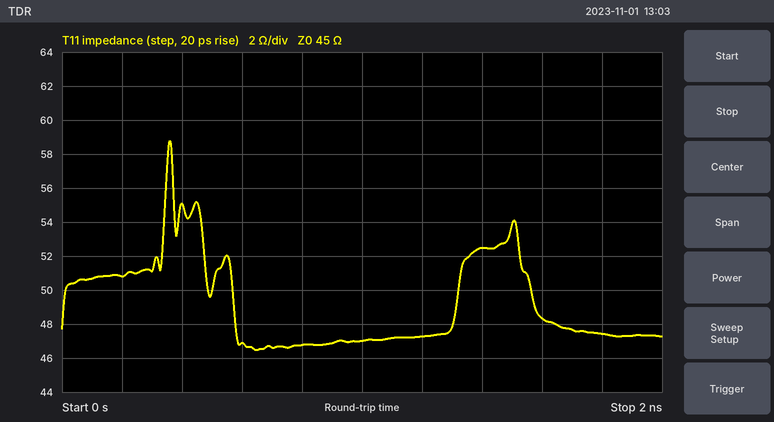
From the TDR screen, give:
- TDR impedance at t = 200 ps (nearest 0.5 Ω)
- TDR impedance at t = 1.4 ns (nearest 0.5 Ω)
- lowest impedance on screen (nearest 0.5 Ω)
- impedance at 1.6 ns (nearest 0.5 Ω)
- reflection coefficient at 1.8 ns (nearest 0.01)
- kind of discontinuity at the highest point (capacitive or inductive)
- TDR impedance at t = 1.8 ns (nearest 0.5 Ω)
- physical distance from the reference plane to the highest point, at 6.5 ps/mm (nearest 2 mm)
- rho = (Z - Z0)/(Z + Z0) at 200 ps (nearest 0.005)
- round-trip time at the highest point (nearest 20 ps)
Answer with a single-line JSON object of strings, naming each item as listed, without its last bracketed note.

{"TDR impedance at t = 200 ps": "51.0 Ω", "TDR impedance at t = 1.4 ns": "52.5 Ω", "lowest impedance on screen": "46.5 Ω", "impedance at 1.6 ns": "48.5 Ω", "reflection coefficient at 1.8 ns": "+0.03", "kind of discontinuity at the highest point": "inductive", "TDR impedance at t = 1.8 ns": "47.5 Ω", "physical distance from the reference plane to the highest point, at 6.5 ps/mm": "28 mm", "rho = (Z - Z0)/(Z + Z0) at 200 ps": "+0.060", "round-trip time at the highest point": "360 ps"}
